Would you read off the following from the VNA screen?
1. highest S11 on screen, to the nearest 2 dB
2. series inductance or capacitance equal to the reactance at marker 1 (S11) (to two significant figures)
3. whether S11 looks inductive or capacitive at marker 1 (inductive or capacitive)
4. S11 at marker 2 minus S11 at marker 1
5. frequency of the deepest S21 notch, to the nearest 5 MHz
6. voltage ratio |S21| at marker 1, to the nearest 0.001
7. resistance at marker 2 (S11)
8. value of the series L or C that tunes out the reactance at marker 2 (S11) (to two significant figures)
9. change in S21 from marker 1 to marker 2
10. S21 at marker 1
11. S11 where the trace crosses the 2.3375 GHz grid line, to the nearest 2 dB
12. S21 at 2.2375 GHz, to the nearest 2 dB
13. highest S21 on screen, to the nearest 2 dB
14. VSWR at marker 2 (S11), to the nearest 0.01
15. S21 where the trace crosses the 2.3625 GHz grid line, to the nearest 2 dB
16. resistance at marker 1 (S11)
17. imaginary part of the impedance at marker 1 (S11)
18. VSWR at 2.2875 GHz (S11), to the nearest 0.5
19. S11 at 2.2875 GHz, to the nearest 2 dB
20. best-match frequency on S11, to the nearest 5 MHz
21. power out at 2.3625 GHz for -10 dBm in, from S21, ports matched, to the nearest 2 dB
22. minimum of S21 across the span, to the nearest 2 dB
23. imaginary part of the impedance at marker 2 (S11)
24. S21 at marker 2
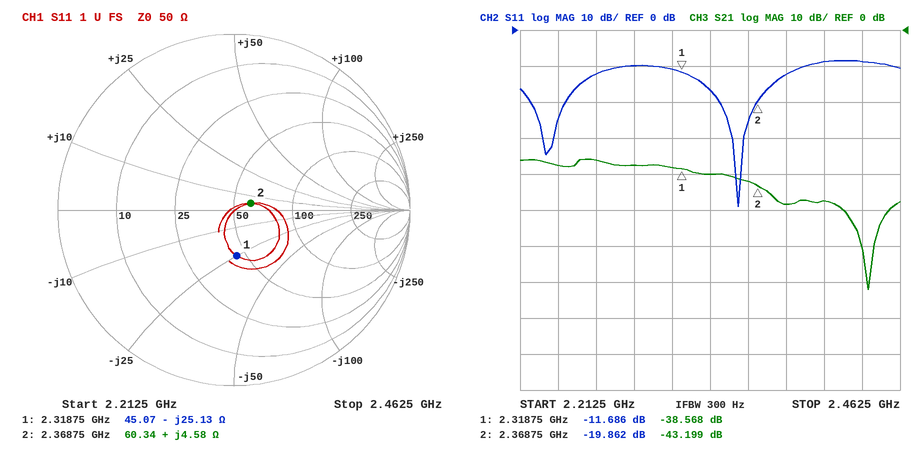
-8 dB
2.7 pF
capacitive
-8.176 dB
2.440 GHz
0.012
60.34 Ω
15 pF
-4.631 dB
-38.568 dB
-16 dB
-38 dB
-36 dB
1.23
-42 dB
45.07 Ω
-25.13 Ω
2.0
-10 dB
2.355 GHz
-52 dBm
-72 dB
+4.58 Ω
-43.199 dB
